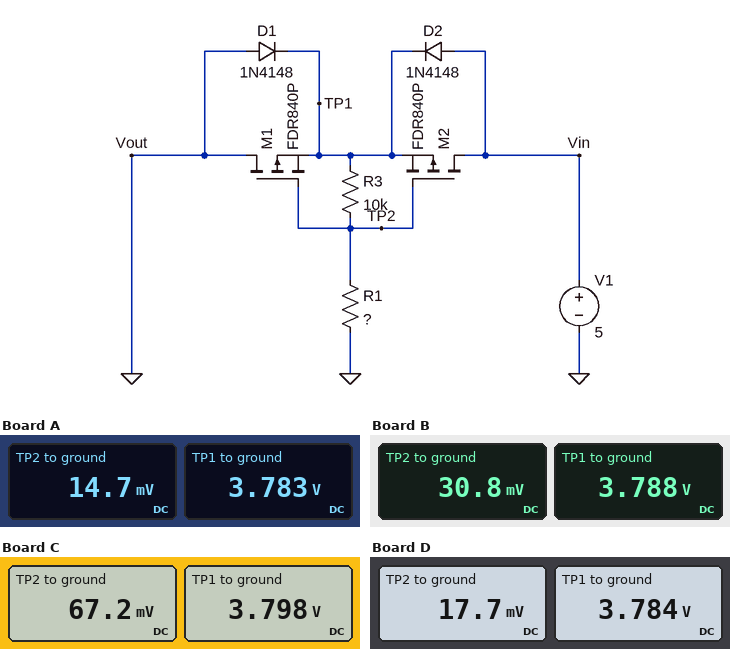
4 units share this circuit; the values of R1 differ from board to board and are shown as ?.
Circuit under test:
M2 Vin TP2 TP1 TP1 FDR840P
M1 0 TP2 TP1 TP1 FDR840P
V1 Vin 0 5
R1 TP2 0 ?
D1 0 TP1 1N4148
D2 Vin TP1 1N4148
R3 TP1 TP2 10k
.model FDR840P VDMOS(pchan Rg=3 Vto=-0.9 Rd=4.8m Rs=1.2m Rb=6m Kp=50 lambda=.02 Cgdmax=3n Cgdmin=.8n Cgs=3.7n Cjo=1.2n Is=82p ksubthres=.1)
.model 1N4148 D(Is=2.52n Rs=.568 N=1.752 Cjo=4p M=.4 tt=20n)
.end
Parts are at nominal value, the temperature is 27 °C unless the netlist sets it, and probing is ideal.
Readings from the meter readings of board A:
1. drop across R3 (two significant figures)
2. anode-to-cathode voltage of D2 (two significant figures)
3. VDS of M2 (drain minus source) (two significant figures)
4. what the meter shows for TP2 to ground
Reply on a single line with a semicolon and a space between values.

3.8 V; 1.2 V; 1.2 V; 14.7 mV
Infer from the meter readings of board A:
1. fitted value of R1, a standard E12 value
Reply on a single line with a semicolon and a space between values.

39 Ω
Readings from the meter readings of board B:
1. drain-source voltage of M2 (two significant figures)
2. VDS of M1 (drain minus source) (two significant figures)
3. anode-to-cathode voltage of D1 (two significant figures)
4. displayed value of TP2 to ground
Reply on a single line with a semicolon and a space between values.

1.2 V; -3.8 V; -3.8 V; 30.8 mV
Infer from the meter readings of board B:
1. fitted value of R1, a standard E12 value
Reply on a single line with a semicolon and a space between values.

82 Ω
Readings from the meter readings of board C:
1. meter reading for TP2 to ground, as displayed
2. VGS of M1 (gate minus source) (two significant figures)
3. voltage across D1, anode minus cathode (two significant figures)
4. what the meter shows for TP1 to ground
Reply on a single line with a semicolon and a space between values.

67.2 mV; -3.7 V; -3.8 V; 3.798 V
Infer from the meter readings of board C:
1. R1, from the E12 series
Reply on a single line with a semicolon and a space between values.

180 Ω
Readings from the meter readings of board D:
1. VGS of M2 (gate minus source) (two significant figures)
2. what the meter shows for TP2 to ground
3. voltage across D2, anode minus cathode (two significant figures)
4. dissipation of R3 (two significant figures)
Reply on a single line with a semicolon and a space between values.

-3.8 V; 17.7 mV; 1.2 V; 1.4 mW
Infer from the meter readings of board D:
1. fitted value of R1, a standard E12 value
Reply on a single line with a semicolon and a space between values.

47 Ω
